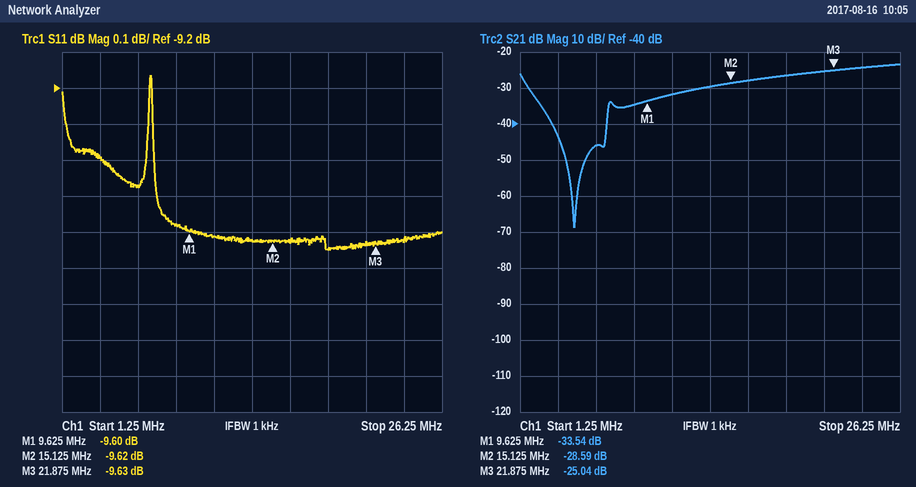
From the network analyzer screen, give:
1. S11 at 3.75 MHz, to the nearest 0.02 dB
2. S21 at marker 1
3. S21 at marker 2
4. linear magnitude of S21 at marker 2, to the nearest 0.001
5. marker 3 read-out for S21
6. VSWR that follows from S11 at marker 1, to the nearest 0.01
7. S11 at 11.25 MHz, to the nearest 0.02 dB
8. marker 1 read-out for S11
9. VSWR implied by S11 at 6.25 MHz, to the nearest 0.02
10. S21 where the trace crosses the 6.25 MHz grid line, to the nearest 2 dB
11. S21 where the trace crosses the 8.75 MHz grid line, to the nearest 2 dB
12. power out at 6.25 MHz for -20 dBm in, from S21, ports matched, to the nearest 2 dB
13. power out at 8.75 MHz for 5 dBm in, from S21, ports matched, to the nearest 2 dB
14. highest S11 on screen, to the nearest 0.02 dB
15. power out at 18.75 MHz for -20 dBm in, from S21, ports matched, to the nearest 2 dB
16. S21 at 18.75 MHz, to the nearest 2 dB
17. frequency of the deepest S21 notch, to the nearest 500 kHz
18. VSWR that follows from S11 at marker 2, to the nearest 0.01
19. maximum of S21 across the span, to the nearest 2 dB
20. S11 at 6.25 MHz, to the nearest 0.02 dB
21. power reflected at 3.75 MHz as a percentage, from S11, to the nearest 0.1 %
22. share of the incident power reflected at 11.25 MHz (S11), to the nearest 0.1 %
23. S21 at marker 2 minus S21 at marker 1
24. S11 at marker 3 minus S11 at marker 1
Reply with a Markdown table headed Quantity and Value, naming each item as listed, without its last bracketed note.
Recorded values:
| Quantity | Value |
|---|---|
| S11 at 3.75 MHz, to the nearest 0.02 dB | -9.40 dB |
| S21 at marker 1 | -33.54 dB |
| S21 at marker 2 | -28.59 dB |
| linear magnitude of S21 at marker 2, to the nearest 0.001 | 0.037 |
| marker 3 read-out for S21 | -25.04 dB |
| VSWR that follows from S11 at marker 1, to the nearest 0.01 | 1.99 |
| S11 at 11.25 MHz, to the nearest 0.02 dB | -9.62 dB |
| marker 1 read-out for S11 | -9.60 dB |
| VSWR implied by S11 at 6.25 MHz, to the nearest 0.02 | 2.02 |
| S21 where the trace crosses the 6.25 MHz grid line, to the nearest 2 dB | -46 dB |
| S21 where the trace crosses the 8.75 MHz grid line, to the nearest 2 dB | -34 dB |
| power out at 6.25 MHz for -20 dBm in, from S21, ports matched, to the nearest 2 dB | -66 dBm |
| power out at 8.75 MHz for 5 dBm in, from S21, ports matched, to the nearest 2 dB | -30 dBm |
| highest S11 on screen, to the nearest 0.02 dB | -9.16 dB |
| power out at 18.75 MHz for -20 dBm in, from S21, ports matched, to the nearest 2 dB | -46 dBm |
| S21 at 18.75 MHz, to the nearest 2 dB | -26 dB |
| frequency of the deepest S21 notch, to the nearest 500 kHz | 5.0 MHz |
| VSWR that follows from S11 at marker 2, to the nearest 0.01 | 1.99 |
| maximum of S21 across the span, to the nearest 2 dB | -24 dB |
| S11 at 6.25 MHz, to the nearest 0.02 dB | -9.48 dB |
| power reflected at 3.75 MHz as a percentage, from S11, to the nearest 0.1 % | 11.5 % |
| share of the incident power reflected at 11.25 MHz (S11), to the nearest 0.1 % | 10.9 % |
| S21 at marker 2 minus S21 at marker 1 | 4.95 dB |
| S11 at marker 3 minus S11 at marker 1 | -0.03 dB |
